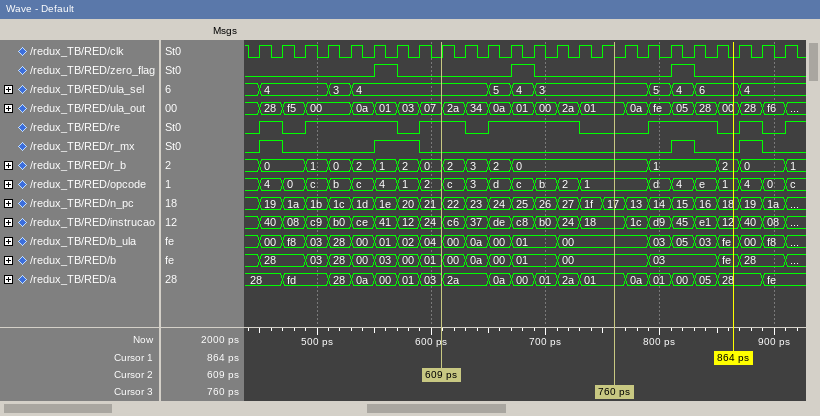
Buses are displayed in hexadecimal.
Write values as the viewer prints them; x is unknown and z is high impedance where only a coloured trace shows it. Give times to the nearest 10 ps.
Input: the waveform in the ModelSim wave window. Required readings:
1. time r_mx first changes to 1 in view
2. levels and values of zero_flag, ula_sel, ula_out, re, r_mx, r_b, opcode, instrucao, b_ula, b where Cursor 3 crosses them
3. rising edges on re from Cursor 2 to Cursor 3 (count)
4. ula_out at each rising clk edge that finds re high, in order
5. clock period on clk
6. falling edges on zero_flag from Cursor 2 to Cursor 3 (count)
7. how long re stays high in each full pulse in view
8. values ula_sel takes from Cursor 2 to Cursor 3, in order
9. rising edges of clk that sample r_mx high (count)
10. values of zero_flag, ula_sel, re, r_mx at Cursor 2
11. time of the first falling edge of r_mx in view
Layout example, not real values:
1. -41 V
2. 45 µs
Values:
1. 450 ps
2. zero_flag=0, ula_sel=3, ula_out=01, re=0, r_mx=0, r_b=0, opcode=1, instrucao=18, b_ula=00, b=00
3. 1
4. 28, 00, 00, 0a, 01, 07, 2a, 0a, 01, 00, 2a, fe, 05, 28, 28
5. 20 ps
6. 1
7. 20 ps, 80 ps, 40 ps, 80 ps, 60 ps, 20 ps
8. 4, 5, 4, 3
9. 5
10. zero_flag=0, ula_sel=4, re=1, r_mx=0
11. 470 ps
